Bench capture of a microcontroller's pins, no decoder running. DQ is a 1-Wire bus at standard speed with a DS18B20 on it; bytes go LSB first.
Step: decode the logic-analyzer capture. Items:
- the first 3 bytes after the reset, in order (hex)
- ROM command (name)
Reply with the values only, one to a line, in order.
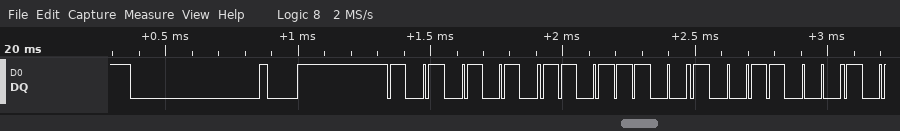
55 3B 19
Match ROM
